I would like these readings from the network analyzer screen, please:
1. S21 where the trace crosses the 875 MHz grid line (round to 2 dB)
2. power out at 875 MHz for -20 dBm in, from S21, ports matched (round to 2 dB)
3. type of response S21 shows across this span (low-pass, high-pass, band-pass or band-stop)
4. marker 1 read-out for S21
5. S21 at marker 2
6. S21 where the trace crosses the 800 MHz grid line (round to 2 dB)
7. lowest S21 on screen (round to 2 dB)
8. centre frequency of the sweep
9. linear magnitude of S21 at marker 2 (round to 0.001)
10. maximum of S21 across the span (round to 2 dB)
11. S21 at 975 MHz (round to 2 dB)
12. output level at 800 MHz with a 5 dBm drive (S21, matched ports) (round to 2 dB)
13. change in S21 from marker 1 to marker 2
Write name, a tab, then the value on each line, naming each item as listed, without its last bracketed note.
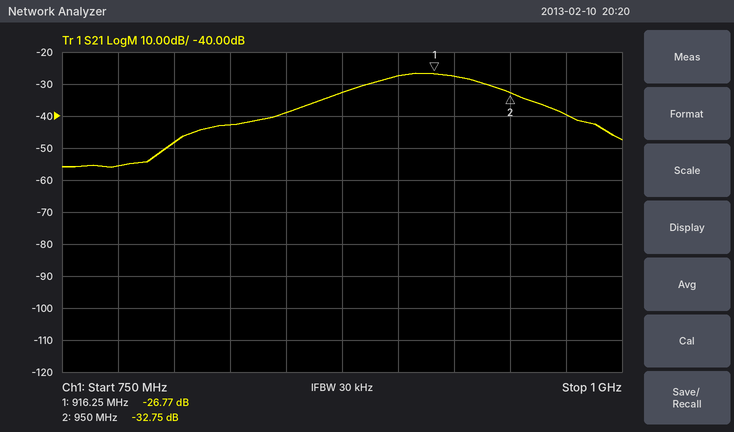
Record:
S21 where the trace crosses the 875 MHz grid line	-32 dB
power out at 875 MHz for -20 dBm in, from S21, ports matched	-52 dBm
type of response S21 shows across this span	band-pass
marker 1 read-out for S21	-26.77 dB
S21 at marker 2	-32.75 dB
S21 where the trace crosses the 800 MHz grid line	-48 dB
lowest S21 on screen	-56 dB
centre frequency of the sweep	875 MHz
linear magnitude of S21 at marker 2	0.023
maximum of S21 across the span	-26 dB
S21 at 975 MHz	-40 dB
output level at 800 MHz with a 5 dBm drive (S21, matched ports)	-44 dBm
change in S21 from marker 1 to marker 2	-5.98 dB
